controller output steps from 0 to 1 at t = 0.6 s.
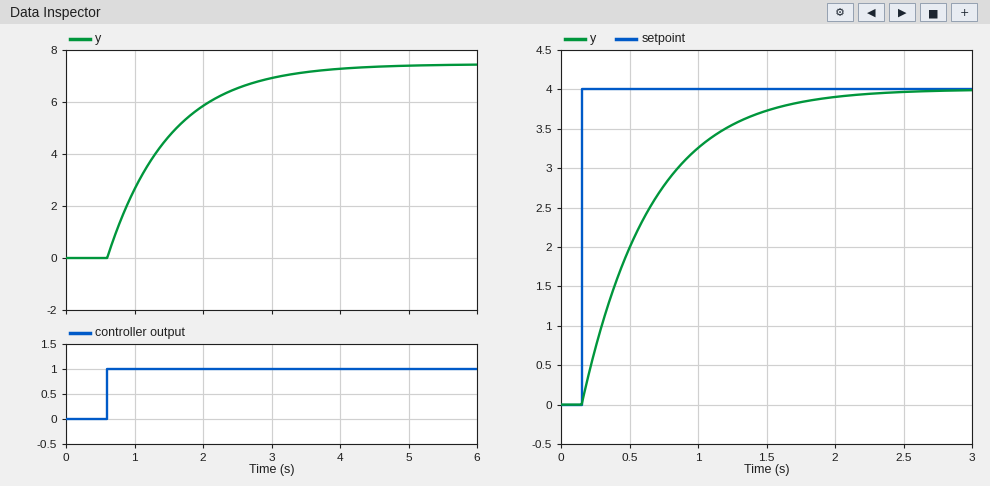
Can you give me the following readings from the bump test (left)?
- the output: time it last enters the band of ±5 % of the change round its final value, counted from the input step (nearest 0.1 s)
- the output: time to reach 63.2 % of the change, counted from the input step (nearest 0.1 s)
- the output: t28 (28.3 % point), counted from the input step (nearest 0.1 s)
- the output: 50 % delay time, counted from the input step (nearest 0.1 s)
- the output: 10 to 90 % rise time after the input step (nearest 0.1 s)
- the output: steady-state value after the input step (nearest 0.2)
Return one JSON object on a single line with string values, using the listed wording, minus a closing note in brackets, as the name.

{"the output: time it last enters the band of ±5 % of the change round its final value, counted from the input step": "2.7 s", "the output: time to reach 63.2 % of the change, counted from the input step": "0.9 s", "the output: t28 (28.3 % point), counted from the input step": "0.3 s", "the output: 50 % delay time, counted from the input step": "0.6 s", "the output: 10 to 90 % rise time after the input step": "2.0 s", "the output: steady-state value after the input step": "7.4"}
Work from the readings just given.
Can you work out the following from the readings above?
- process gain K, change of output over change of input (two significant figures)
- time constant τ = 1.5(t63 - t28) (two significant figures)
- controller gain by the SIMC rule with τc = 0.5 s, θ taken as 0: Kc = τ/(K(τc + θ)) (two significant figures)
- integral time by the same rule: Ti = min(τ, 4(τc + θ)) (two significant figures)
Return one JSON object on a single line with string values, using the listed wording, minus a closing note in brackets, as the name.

{"process gain K, change of output over change of input": "7.4", "time constant τ = 1.5(t63 - t28)": "0.90 s", "controller gain by the SIMC rule with τc = 0.5 s, θ taken as 0: Kc = τ/(K(τc + θ))": "0.24", "integral time by the same rule: Ti = min(τ, 4(τc + θ))": "0.90 s"}
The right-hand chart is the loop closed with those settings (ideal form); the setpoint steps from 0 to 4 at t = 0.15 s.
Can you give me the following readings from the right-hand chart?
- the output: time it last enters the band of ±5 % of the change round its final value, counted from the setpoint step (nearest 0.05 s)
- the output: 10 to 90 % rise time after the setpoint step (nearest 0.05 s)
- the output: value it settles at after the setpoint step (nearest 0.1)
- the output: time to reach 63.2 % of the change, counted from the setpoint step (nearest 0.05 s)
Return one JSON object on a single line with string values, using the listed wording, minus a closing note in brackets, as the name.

{"the output: time it last enters the band of ±5 % of the change round its final value, counted from the setpoint step": "1.50 s", "the output: 10 to 90 % rise time after the setpoint step": "1.10 s", "the output: value it settles at after the setpoint step": "4.0", "the output: time to reach 63.2 % of the change, counted from the setpoint step": "0.50 s"}
